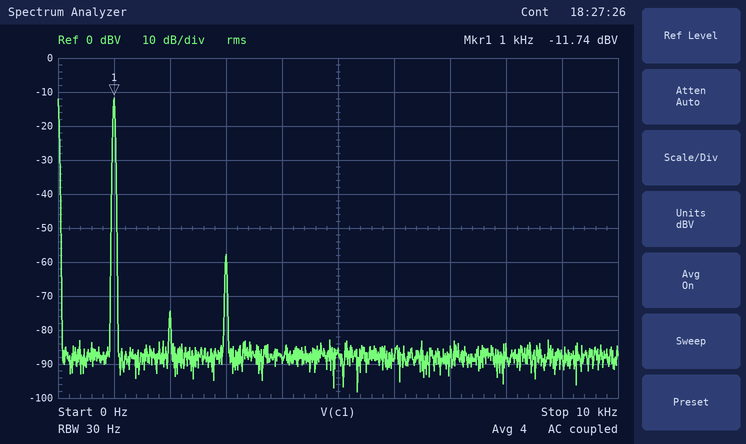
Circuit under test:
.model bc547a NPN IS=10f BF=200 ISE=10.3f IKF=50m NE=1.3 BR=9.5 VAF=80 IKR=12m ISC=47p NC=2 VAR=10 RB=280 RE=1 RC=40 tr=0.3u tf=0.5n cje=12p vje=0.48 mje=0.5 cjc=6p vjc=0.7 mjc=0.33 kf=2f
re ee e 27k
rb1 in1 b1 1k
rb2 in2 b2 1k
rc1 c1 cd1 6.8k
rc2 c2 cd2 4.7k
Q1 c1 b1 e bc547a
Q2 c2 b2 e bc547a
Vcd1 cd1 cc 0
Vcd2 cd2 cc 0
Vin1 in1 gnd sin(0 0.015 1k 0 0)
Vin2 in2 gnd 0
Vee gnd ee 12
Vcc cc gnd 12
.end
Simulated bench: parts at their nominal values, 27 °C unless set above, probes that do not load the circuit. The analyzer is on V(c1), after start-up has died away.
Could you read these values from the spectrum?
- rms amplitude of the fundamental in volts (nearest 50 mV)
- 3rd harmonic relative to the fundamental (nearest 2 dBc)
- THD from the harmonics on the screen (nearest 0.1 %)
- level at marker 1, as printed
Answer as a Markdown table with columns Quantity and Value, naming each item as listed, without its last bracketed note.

| Quantity | Value |
|---|---|
| rms amplitude of the fundamental in volts | 250 mV |
| 3rd harmonic relative to the fundamental | -46 dBc |
| THD from the harmonics on the screen | 0.5 % |
| level at marker 1, as printed | -11.74 dBV |
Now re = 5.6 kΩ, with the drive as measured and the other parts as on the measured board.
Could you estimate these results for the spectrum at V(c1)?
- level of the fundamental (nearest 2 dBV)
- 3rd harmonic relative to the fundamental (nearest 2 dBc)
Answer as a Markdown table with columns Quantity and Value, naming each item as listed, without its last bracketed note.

| Quantity | Value |
|---|---|
| level of the fundamental | 0 dBV |
| 3rd harmonic relative to the fundamental | -54 dBc |
